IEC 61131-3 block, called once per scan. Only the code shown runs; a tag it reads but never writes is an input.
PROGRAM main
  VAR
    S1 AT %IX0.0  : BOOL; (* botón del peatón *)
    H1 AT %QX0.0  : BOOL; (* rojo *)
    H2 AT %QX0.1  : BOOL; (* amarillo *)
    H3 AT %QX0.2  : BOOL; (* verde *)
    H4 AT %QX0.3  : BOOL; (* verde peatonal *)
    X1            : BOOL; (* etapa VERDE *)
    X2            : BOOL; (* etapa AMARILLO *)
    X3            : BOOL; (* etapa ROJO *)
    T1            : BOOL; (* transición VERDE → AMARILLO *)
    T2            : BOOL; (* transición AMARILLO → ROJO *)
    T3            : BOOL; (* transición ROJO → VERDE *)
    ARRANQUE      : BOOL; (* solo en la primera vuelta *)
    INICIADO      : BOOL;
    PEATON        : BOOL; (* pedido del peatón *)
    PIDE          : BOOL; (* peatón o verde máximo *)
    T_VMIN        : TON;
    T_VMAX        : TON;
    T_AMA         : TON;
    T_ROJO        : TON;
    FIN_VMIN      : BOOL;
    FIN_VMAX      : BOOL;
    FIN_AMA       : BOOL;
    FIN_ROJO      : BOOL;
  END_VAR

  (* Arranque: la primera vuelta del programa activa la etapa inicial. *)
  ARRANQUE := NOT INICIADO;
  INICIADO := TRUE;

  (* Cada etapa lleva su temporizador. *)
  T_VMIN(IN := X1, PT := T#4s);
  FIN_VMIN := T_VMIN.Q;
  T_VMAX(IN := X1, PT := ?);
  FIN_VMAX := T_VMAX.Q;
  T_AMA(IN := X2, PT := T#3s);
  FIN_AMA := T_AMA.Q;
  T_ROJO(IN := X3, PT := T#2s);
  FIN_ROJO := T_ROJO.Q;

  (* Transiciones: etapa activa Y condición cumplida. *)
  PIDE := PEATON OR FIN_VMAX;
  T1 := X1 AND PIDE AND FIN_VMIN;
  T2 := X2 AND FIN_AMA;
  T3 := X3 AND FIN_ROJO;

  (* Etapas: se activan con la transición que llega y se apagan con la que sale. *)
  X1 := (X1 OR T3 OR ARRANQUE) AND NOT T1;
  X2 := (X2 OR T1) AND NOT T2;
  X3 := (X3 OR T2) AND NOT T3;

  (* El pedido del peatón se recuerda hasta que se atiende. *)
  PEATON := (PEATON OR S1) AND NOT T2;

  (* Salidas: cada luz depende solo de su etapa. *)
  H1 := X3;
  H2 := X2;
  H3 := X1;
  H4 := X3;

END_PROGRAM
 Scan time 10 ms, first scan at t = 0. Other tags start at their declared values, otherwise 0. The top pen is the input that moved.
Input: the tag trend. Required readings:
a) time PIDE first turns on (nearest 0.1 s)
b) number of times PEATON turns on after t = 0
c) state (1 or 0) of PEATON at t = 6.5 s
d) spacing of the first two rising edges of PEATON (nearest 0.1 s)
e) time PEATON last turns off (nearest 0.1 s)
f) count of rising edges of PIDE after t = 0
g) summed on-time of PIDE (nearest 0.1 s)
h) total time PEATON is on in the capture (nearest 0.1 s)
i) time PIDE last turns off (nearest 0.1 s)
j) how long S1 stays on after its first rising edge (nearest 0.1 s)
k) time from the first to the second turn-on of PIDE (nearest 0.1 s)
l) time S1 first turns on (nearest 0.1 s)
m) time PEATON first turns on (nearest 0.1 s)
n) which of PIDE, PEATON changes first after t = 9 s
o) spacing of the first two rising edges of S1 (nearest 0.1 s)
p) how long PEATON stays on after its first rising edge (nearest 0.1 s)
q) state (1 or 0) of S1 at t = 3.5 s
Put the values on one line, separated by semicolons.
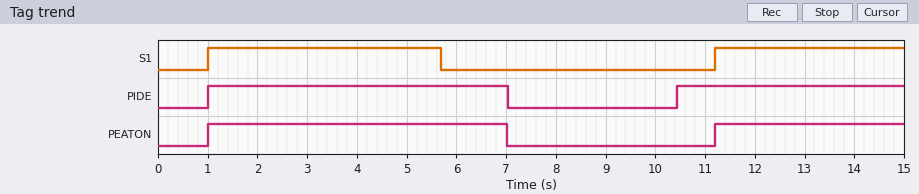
1.0 s; 2; 1; 10.2 s; 7.0 s; 2; 10.6 s; 9.8 s; 7.0 s; 4.7 s; 9.4 s; 1.0 s; 1.0 s; PIDE; 10.2 s; 6.0 s; 1
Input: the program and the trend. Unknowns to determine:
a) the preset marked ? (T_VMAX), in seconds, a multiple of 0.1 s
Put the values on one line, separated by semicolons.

1.4 s
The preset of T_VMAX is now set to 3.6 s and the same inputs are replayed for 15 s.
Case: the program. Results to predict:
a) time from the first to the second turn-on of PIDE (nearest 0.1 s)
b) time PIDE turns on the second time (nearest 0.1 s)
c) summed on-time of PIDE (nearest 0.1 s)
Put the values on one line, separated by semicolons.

10.2 s; 11.2 s; 9.8 s
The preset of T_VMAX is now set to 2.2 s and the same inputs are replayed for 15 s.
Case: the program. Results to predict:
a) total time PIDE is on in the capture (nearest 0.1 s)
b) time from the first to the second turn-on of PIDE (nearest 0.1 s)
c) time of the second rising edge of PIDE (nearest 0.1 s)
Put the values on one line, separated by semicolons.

9.8 s; 10.2 s; 11.2 s
